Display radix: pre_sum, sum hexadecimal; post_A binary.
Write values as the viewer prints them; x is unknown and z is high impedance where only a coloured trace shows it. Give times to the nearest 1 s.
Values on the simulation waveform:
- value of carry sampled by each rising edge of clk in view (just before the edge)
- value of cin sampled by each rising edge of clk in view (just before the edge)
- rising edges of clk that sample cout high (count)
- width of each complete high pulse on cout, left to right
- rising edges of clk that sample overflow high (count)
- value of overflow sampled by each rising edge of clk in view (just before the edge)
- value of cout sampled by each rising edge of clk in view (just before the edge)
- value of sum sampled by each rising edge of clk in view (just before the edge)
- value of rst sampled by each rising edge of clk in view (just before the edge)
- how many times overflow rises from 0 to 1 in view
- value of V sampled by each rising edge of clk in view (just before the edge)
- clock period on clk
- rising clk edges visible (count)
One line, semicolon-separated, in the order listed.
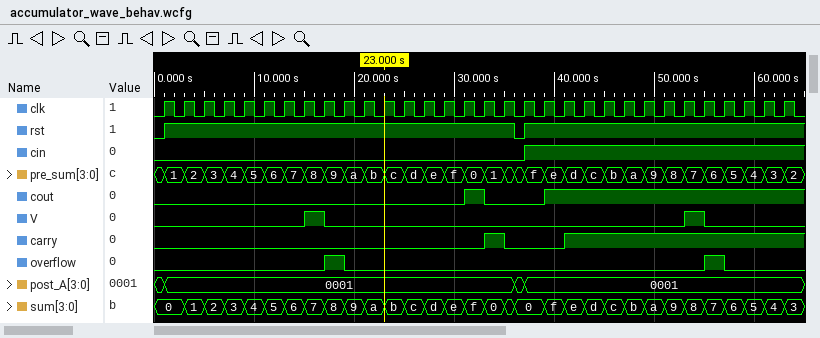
0 0 0 0 0 0 0 0 0 0 0 0 0 0 0 0 0 1 0 0 0 1 1 1 1 1 1 1 1 1 1 1; 0 0 0 0 0 0 0 0 0 0 0 0 0 0 0 0 0 0 0 1 1 1 1 1 1 1 1 1 1 1 1 1; 13; 2 s; 2; 0 0 0 0 0 0 0 0 0 1 0 0 0 0 0 0 0 0 0 0 0 0 0 0 0 0 0 0 1 0 0 0; 0 0 0 0 0 0 0 0 0 0 0 0 0 0 0 0 1 0 0 0 1 1 1 1 1 1 1 1 1 1 1 1; 0, 0, 1, 2, 3, 4, 5, 6, 7, 8, 9, a, b, c, d, e, f, 0, 0, 0, f, e, d, c, b, a, 9, 8, 7, 6, 5, 4; 0 1 1 1 1 1 1 1 1 1 1 1 1 1 1 1 1 1 0 1 1 1 1 1 1 1 1 1 1 1 1 1; 2; 0 0 0 0 0 0 0 0 1 0 0 0 0 0 0 0 0 0 0 0 0 0 0 0 0 0 0 1 0 0 0 0; 2 s; 32
